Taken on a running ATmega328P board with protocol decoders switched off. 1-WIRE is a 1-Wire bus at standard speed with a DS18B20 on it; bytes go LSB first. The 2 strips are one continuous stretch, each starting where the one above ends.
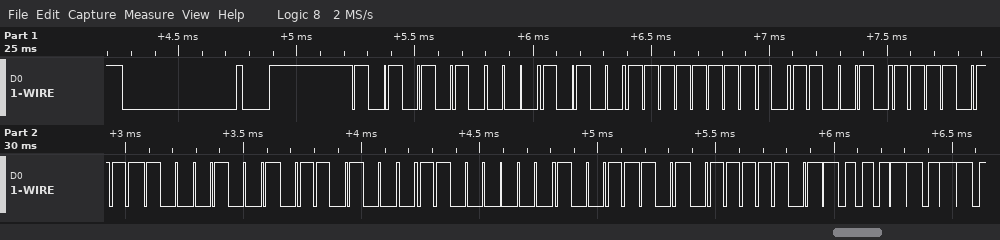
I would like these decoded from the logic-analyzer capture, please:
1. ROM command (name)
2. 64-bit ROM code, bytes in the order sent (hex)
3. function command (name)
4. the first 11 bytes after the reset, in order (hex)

Match ROM
28 FF 4D EF 91 16 03 B9
Read Scratchpad
55 28 FF 4D EF 91 16 03 B9 BE B1
